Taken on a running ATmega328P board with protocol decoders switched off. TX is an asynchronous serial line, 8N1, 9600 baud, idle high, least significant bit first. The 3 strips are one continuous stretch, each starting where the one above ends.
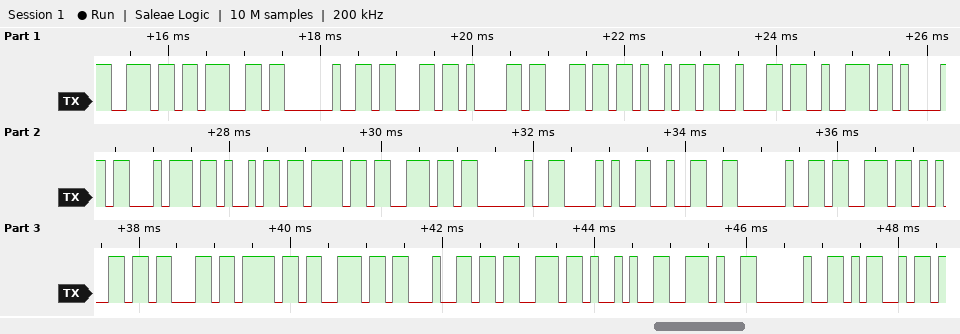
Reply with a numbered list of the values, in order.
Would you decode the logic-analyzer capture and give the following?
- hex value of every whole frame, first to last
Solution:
1. 6E 67 20 63 61 6C 69 62 72 61 74 69 6F 6E 20 28 32 20 73 65 63 6F 6E 64 73 29 2E 20 4D
